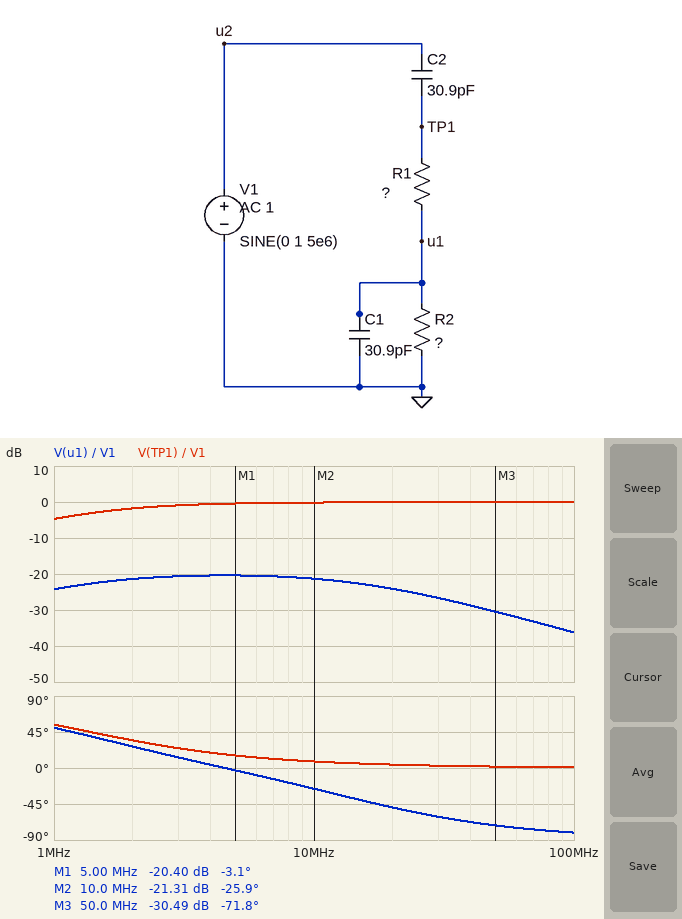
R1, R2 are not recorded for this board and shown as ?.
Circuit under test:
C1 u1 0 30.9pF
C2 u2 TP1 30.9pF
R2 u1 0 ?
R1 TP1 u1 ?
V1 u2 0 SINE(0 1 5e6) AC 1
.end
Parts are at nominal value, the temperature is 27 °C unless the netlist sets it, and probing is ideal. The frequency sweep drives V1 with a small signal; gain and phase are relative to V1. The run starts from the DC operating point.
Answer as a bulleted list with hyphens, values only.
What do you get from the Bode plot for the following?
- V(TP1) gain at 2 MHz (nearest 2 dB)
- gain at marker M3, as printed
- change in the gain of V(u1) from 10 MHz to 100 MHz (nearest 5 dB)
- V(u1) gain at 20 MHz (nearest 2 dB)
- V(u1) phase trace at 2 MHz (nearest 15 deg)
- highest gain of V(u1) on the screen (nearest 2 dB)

- -2 dB
- -30.49 dB
- -15 dB
- -24 dB
- 30 deg
- -20 dB
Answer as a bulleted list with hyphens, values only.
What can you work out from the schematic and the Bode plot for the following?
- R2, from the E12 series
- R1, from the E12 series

- 390 Ω
- 3.3 kΩ
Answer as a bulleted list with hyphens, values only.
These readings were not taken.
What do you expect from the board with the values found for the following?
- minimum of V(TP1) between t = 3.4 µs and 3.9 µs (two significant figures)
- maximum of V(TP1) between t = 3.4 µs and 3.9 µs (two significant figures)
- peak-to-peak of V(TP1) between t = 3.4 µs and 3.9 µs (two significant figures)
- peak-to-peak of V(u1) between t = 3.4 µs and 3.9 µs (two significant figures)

- -950 mV
- 950 mV
- 1.9 V
- 190 mV
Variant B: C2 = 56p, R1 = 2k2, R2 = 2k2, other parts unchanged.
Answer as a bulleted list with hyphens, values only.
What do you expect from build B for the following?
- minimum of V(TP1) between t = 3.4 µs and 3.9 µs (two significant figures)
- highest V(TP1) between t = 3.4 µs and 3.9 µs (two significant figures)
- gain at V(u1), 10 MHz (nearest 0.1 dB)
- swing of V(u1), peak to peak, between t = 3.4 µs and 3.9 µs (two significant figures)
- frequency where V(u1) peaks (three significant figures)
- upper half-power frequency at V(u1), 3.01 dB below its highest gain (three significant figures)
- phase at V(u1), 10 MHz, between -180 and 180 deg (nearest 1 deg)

- -920 mV
- 920 mV
- -13.7 dB
- 630 mV
- 1.74 MHz
- 6.44 MHz
- -58 deg
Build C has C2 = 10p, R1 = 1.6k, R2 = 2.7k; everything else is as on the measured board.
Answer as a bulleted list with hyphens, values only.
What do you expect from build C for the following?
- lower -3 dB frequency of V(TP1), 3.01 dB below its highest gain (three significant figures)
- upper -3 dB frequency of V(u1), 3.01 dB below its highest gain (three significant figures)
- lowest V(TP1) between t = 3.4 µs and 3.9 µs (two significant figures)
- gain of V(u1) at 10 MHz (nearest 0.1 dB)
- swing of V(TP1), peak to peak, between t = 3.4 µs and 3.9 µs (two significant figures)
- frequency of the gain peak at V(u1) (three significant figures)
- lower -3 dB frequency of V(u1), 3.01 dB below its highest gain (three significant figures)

- 11.8 MHz
- 16.2 MHz
- -470 mV
- -14.5 dB
- 950 mV
- 4.36 MHz
- 1.17 MHz
